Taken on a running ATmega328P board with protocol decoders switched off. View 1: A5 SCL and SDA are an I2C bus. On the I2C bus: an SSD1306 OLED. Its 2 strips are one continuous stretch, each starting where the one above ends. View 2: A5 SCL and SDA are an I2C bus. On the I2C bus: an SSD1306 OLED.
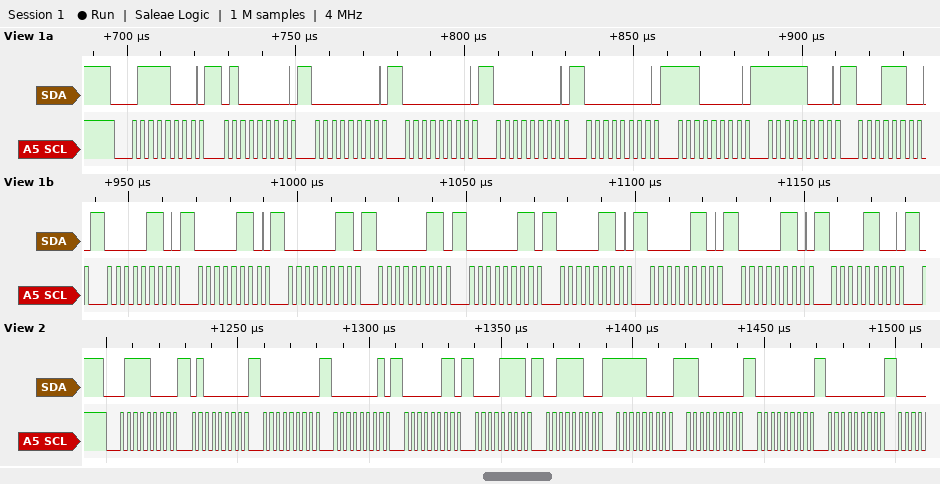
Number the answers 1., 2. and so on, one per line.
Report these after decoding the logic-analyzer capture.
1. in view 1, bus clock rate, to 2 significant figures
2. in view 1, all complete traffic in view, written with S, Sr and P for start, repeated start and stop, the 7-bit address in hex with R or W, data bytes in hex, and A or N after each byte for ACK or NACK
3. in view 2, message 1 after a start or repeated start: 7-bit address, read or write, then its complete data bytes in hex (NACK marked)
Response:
1. 400 kHz
2. S 3CW A 40 A 00 A 00 A 00 A 00 A E0 A F8 A 1C A 06 A 06 A 03 A 03 A 03 A 06 A 06 A 06 A 0C A
3. 0x3C write: 40 00 01 03 0F 3C F8 C0 00 00
